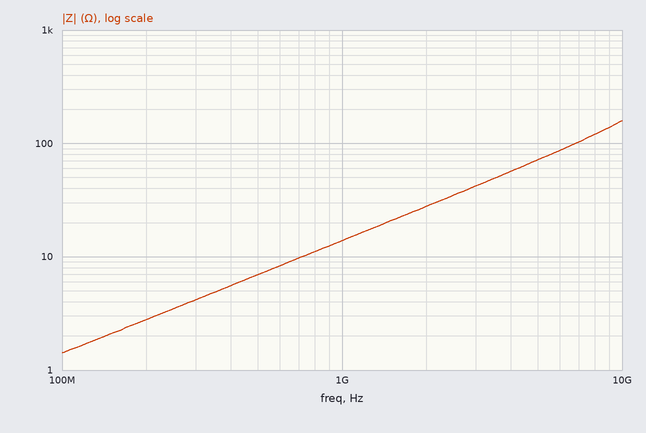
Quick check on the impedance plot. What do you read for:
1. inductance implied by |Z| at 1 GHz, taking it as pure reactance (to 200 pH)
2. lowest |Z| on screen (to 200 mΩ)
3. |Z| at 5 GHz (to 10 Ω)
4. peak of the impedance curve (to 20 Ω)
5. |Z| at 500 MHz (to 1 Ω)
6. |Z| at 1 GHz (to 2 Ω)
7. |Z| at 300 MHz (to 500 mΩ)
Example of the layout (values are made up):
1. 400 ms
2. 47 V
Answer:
1. 2.2 nH
2. 1.4 Ω
3. 70 Ω
4. 160 Ω
5. 7 Ω
6. 14 Ω
7. 4.0 Ω
